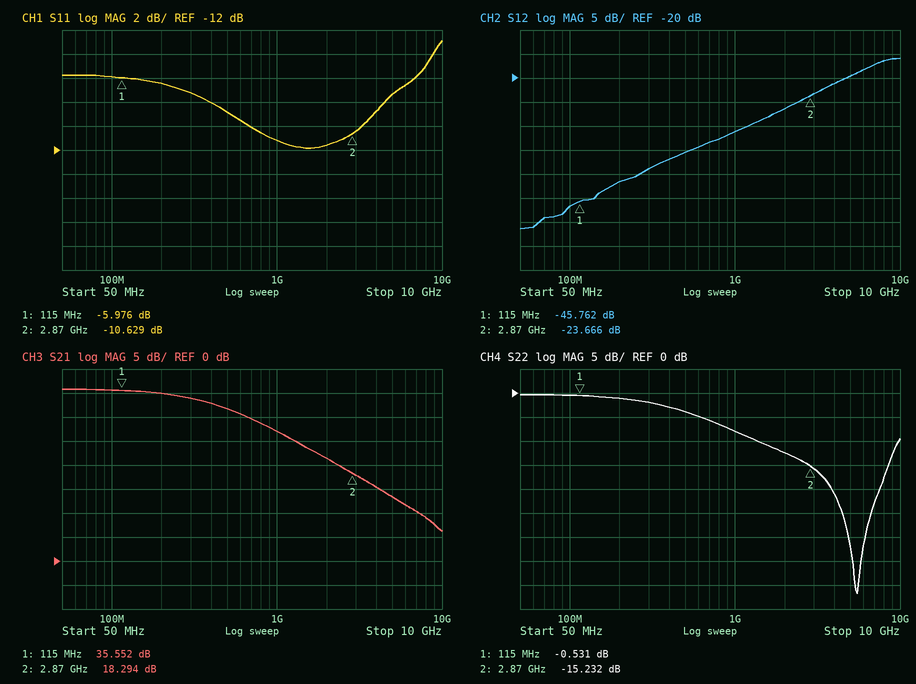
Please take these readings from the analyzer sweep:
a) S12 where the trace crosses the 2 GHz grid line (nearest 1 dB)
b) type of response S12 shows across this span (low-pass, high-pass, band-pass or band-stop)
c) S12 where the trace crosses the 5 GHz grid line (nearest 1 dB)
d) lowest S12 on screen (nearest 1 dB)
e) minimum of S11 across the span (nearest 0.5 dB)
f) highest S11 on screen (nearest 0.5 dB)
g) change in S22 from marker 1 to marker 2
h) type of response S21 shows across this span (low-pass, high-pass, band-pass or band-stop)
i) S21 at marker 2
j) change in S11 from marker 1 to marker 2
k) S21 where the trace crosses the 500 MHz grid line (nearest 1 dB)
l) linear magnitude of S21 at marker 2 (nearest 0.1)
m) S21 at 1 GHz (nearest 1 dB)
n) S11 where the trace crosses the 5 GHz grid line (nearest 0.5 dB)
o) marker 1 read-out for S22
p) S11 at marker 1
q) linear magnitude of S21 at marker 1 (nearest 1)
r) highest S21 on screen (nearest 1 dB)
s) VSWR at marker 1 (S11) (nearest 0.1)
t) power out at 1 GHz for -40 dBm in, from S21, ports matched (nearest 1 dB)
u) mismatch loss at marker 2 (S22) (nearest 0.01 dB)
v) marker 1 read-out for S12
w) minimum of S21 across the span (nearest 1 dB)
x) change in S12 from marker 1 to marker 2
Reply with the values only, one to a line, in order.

-26 dB
high-pass
-20 dB
-51 dB
-12.0 dB
-3.0 dB
-14.701 dB
low-pass
18.294 dB
-4.653 dB
32 dB
8.2
27 dB
-7.5 dB
-0.531 dB
-5.976 dB
60
36 dB
3.0
-13 dBm
0.13 dB
-45.762 dB
6 dB
22.096 dB
